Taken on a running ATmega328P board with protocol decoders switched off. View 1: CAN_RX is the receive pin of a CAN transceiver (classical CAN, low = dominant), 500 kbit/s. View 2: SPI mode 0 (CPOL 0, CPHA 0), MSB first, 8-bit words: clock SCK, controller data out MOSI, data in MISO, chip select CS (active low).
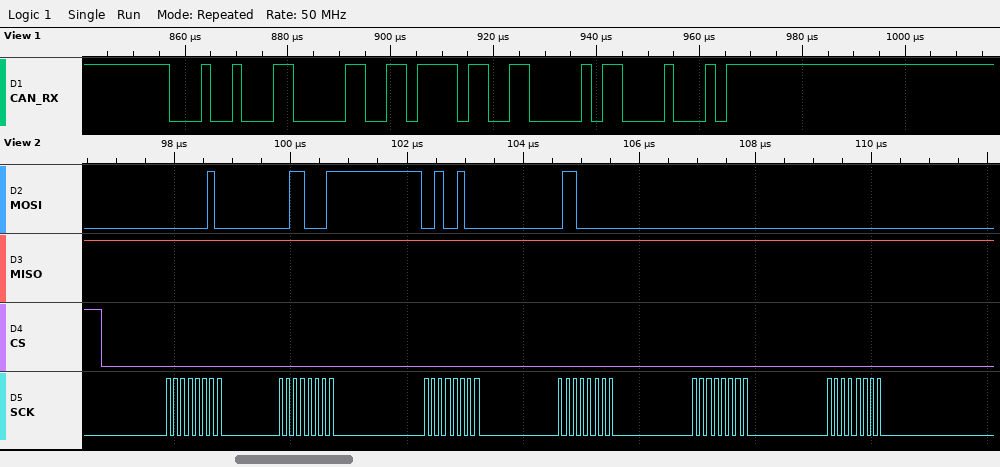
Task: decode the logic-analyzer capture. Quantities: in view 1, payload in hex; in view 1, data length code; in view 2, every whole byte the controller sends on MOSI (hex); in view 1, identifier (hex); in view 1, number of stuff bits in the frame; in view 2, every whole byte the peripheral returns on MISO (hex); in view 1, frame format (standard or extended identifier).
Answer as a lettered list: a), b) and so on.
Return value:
a) 6F 66
b) 2
c) 0x02 0x31 0x24 0x60 0x00 0x00
d) 0x123
e) 2
f) 0xFF 0xFF 0xFF 0xFF 0xFF 0xFF
g) standard
